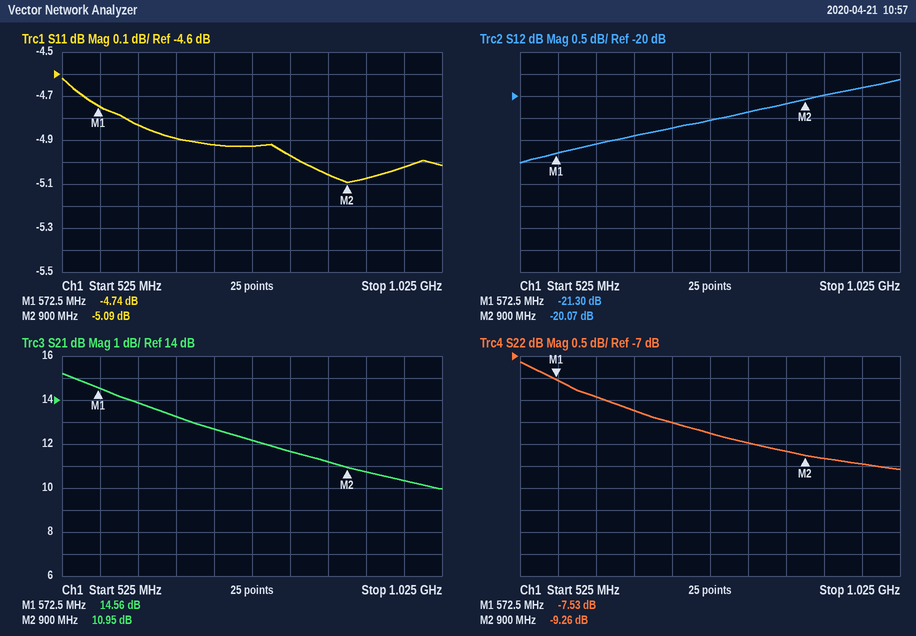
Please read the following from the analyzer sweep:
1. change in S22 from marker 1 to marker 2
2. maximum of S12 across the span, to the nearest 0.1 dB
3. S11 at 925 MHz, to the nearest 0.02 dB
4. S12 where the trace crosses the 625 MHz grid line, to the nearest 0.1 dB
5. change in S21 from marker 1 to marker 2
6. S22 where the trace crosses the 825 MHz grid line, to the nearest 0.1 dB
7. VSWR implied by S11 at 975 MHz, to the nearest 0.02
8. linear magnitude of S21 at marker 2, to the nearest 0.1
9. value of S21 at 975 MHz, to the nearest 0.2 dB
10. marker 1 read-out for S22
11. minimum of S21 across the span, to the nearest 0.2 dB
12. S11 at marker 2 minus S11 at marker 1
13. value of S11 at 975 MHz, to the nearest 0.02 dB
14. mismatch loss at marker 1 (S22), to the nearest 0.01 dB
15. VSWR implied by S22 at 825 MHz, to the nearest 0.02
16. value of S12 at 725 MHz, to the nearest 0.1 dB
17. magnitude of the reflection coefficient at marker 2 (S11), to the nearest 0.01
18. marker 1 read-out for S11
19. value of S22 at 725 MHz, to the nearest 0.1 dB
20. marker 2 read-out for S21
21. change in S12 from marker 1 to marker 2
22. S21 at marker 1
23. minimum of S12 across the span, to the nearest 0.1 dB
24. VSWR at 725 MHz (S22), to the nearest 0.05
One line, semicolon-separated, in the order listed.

-1.73 dB; -19.6 dB; -5.08 dB; -21.1 dB; -3.61 dB; -9.0 dB; 3.56; 3.5; 10.4 dB; -7.53 dB; 10.0 dB; -0.35 dB; -5.02 dB; 0.84 dB; 2.10; -20.7 dB; 0.56; -4.74 dB; -8.5 dB; 10.95 dB; 1.23 dB; 14.56 dB; -21.5 dB; 2.20
